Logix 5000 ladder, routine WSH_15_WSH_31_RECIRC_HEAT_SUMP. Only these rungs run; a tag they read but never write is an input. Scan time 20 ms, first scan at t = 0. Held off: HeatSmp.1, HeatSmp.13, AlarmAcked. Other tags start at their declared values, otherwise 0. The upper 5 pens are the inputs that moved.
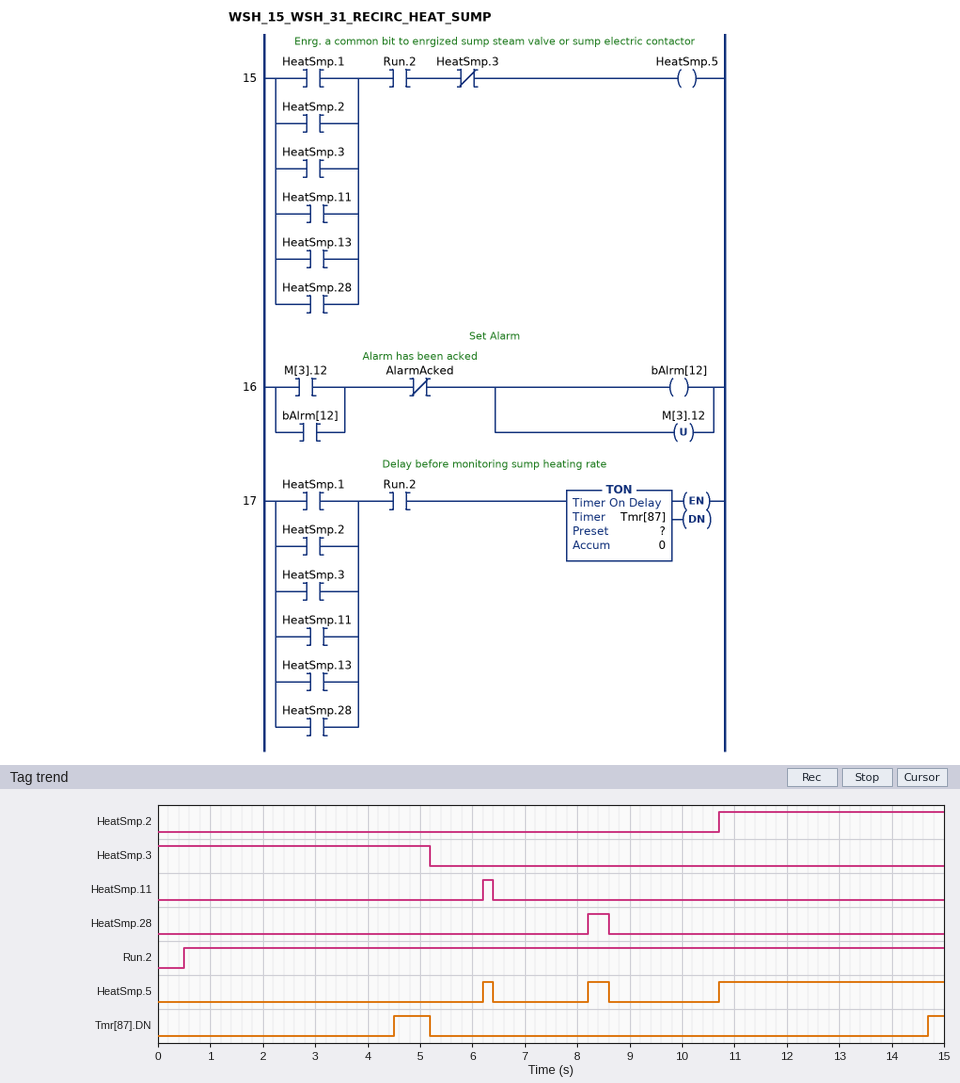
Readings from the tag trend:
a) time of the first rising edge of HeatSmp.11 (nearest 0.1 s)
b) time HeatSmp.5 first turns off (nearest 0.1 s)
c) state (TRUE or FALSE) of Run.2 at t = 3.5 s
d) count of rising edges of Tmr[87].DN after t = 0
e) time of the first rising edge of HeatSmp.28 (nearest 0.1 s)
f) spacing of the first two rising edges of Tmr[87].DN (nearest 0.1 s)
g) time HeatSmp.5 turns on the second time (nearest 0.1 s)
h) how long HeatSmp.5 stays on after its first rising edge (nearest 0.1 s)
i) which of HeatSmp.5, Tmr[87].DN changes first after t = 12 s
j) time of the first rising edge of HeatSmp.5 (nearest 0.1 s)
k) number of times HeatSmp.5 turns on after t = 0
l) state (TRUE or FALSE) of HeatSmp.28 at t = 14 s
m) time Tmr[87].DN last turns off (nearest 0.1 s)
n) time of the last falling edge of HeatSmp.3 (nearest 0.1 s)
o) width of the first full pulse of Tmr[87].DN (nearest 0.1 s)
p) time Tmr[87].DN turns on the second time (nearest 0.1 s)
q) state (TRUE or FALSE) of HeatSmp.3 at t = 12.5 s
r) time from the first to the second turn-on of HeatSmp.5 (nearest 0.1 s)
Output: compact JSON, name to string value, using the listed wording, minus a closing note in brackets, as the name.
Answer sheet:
{"time of the first rising edge of HeatSmp.11": "6.2 s", "time HeatSmp.5 first turns off": "6.4 s", "state (TRUE or FALSE) of Run.2 at t = 3.5 s": "TRUE", "count of rising edges of Tmr[87].DN after t = 0": "2", "time of the first rising edge of HeatSmp.28": "8.2 s", "spacing of the first two rising edges of Tmr[87].DN": "10.2 s", "time HeatSmp.5 turns on the second time": "8.2 s", "how long HeatSmp.5 stays on after its first rising edge": "0.2 s", "which of HeatSmp.5, Tmr[87].DN changes first after t = 12 s": "Tmr[87].DN", "time of the first rising edge of HeatSmp.5": "6.2 s", "number of times HeatSmp.5 turns on after t = 0": "3", "state (TRUE or FALSE) of HeatSmp.28 at t = 14 s": "FALSE", "time Tmr[87].DN last turns off": "5.2 s", "time of the last falling edge of HeatSmp.3": "5.2 s", "width of the first full pulse of Tmr[87].DN": "0.7 s", "time Tmr[87].DN turns on the second time": "14.7 s", "state (TRUE or FALSE) of HeatSmp.3 at t = 12.5 s": "FALSE", "time from the first to the second turn-on of HeatSmp.5": "2.0 s"}
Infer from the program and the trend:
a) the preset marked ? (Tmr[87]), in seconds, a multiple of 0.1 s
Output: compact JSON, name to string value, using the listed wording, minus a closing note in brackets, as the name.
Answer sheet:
{"the preset marked ? (Tmr[87]), in seconds, a multiple of 0.1 s": "4.0 s"}
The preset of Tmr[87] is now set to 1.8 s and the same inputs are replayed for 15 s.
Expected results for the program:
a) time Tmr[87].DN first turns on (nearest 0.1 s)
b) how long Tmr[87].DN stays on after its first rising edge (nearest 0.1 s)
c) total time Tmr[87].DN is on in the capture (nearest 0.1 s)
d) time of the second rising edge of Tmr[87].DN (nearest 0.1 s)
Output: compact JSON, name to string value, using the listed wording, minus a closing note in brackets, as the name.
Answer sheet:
{"time Tmr[87].DN first turns on": "2.3 s", "how long Tmr[87].DN stays on after its first rising edge": "2.9 s", "total time Tmr[87].DN is on in the capture": "5.4 s", "time of the second rising edge of Tmr[87].DN": "12.5 s"}
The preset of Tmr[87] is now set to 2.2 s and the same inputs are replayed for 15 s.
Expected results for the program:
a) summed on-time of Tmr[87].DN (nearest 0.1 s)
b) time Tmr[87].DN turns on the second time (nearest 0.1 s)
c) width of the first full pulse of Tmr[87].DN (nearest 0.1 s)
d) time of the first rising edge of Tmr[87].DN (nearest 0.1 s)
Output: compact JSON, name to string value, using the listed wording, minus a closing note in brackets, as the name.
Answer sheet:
{"summed on-time of Tmr[87].DN": "4.6 s", "time Tmr[87].DN turns on the second time": "12.9 s", "width of the first full pulse of Tmr[87].DN": "2.5 s", "time of the first rising edge of Tmr[87].DN": "2.7 s"}
